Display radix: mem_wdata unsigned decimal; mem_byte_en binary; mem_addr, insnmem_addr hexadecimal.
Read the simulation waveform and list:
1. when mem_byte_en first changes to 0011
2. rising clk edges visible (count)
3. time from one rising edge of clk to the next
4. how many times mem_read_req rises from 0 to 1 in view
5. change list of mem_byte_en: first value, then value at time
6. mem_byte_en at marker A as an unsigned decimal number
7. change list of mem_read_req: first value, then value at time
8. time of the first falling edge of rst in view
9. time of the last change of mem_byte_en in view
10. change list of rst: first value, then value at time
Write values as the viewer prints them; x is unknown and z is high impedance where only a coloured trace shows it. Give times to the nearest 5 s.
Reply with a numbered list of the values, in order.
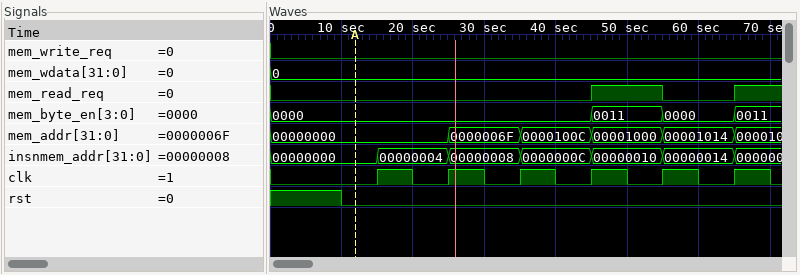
1. 45 s
2. 6
3. 10 s
4. 2
5. 0000, 0011 at 45 s, 0000 at 55 s, 0011 at 65 s
6. 0
7. 0, 1 at 45 s, 0 at 55 s, 1 at 65 s
8. 10 s
9. 65 s
10. 1, 0 at 10 s
